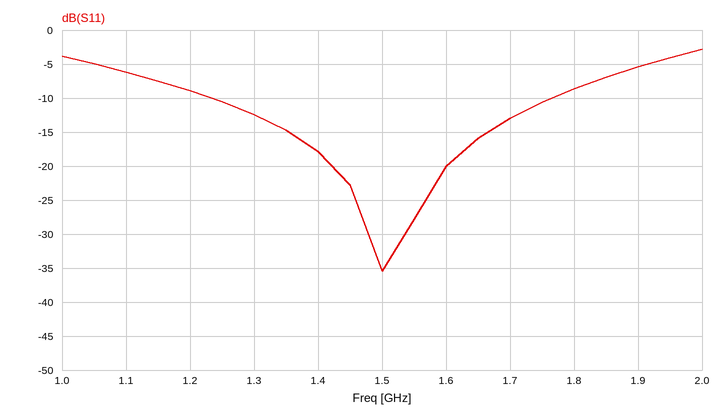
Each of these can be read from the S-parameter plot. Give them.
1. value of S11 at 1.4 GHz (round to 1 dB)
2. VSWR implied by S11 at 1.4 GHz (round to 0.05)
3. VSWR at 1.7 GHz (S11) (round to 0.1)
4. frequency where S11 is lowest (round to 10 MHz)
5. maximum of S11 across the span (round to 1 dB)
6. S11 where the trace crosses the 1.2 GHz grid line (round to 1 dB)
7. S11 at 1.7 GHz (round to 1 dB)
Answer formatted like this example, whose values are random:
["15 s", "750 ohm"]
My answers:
["-18 dB", "1.30", "1.6", "1.50 GHz", "-3 dB", "-9 dB", "-13 dB"]
